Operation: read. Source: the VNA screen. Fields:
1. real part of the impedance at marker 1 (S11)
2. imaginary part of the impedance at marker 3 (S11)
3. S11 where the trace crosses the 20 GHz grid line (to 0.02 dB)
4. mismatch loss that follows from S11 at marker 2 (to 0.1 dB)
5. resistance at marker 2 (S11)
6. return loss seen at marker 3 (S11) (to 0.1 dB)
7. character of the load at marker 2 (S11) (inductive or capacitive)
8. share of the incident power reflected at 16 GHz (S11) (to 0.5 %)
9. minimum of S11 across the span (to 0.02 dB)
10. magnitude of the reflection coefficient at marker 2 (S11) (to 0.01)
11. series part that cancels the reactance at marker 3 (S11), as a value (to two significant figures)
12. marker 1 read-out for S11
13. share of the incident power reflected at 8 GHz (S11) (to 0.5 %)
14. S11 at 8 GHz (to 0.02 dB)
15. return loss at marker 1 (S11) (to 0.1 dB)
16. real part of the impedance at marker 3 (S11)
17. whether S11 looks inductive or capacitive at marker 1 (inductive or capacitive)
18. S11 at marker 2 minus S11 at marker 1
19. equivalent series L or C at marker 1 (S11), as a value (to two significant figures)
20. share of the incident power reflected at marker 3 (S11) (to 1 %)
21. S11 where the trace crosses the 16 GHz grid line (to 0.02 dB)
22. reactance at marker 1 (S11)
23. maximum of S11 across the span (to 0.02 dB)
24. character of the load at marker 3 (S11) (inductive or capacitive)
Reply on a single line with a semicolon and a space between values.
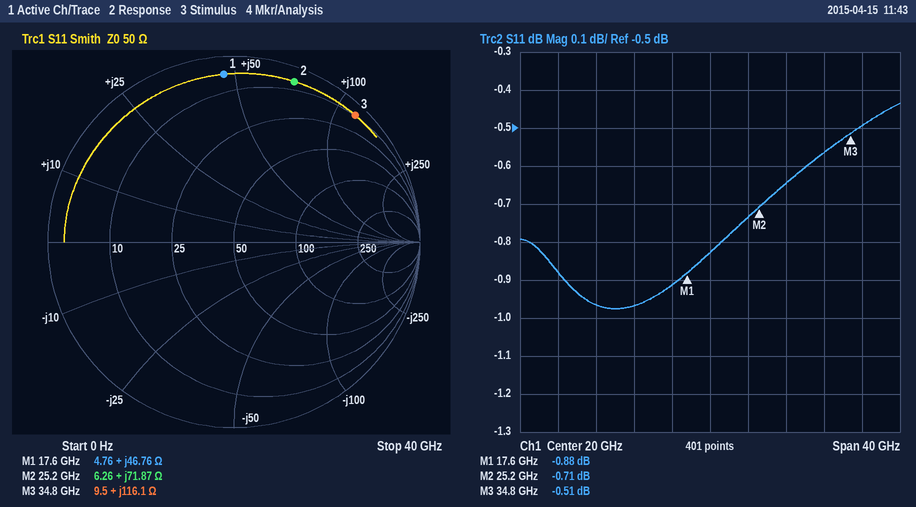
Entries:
4.76 Ω; +116.1 Ω; -0.82 dB; 8.2 dB; 6.26 Ω; 0.5 dB; inductive; 81.0 %; -0.98 dB; 0.92; 39 fF; -0.88 dB; 80.0 %; -0.96 dB; 0.9 dB; 9.5 Ω; inductive; 0.17 dB; 420 pH; 89 %; -0.92 dB; +46.76 Ω; -0.44 dB; inductive
